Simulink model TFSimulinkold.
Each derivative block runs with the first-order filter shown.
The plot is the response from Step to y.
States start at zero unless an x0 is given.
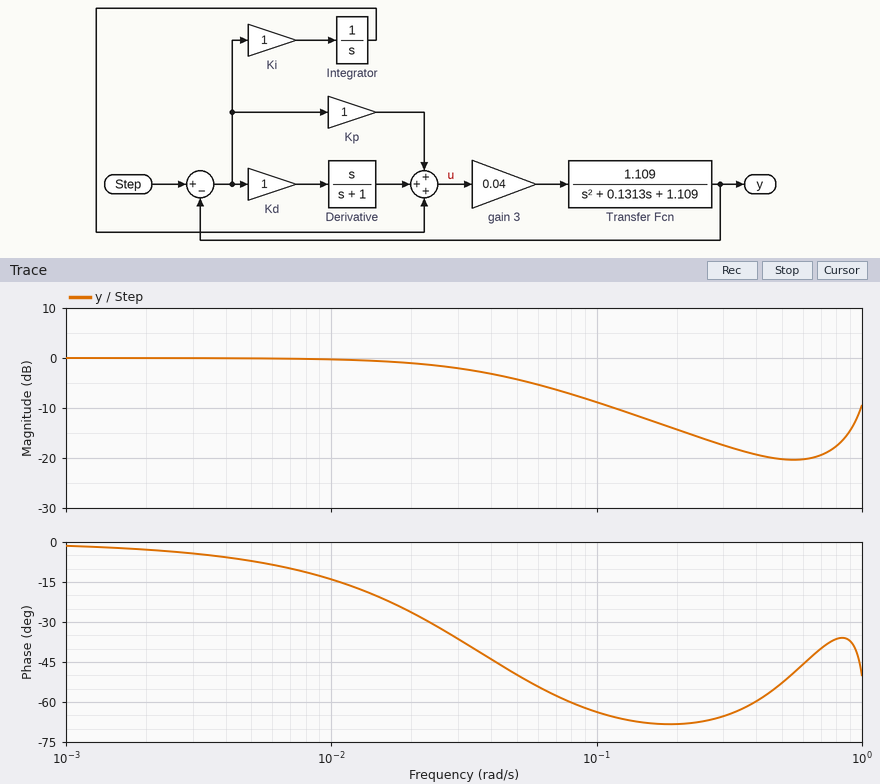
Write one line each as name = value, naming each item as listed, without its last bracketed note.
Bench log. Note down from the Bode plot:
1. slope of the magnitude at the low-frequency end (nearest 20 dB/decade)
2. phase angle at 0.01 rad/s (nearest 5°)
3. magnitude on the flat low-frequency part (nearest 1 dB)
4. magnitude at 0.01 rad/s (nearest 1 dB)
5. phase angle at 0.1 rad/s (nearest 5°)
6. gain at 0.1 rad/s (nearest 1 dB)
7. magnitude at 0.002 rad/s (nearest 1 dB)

slope of the magnitude at the low-frequency end = 0 dB/decade
phase angle at 0.01 rad/s = -15°
magnitude on the flat low-frequency part = 0 dB
magnitude at 0.01 rad/s = 0 dB
phase angle at 0.1 rad/s = -65°
gain at 0.1 rad/s = -9 dB
magnitude at 0.002 rad/s = 0 dB
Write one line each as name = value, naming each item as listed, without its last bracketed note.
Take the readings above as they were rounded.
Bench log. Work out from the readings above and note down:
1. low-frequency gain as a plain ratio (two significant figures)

low-frequency gain as a plain ratio = 1.0
